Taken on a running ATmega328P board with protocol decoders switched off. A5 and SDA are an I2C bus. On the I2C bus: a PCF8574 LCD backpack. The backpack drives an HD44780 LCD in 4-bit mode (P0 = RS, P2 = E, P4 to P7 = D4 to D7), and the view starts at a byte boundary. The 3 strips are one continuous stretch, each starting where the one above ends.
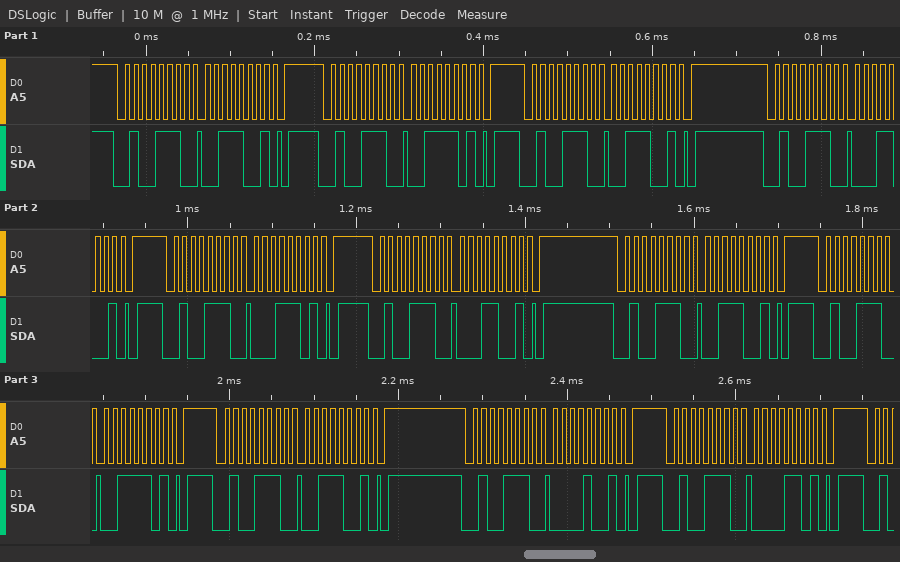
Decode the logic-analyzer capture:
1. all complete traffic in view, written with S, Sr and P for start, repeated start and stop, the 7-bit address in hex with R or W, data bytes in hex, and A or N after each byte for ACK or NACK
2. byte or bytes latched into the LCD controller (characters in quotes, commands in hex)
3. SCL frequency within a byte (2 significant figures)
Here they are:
S 27W A 39 A P S 27W A 3D A P S 27W A 39 A P S 27W A 19 A P S 27W A 1D A P S 27W A 19 A P S 27W A 39 A P S 27W A 3D A P S 27W A 39 A P S 27W A 09 A P S 27W A 0D A P
'1'
100 kHz
